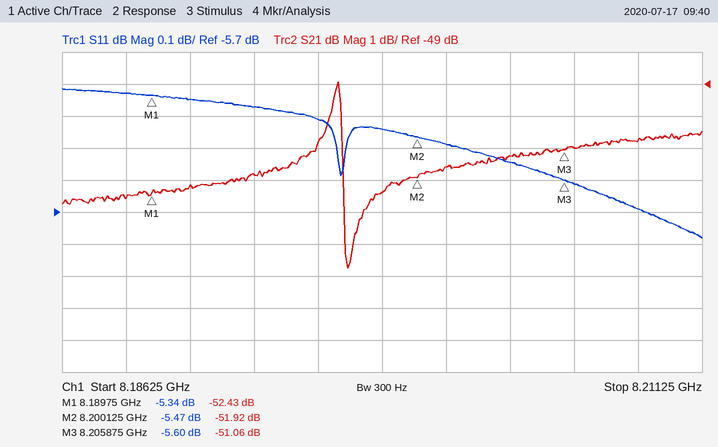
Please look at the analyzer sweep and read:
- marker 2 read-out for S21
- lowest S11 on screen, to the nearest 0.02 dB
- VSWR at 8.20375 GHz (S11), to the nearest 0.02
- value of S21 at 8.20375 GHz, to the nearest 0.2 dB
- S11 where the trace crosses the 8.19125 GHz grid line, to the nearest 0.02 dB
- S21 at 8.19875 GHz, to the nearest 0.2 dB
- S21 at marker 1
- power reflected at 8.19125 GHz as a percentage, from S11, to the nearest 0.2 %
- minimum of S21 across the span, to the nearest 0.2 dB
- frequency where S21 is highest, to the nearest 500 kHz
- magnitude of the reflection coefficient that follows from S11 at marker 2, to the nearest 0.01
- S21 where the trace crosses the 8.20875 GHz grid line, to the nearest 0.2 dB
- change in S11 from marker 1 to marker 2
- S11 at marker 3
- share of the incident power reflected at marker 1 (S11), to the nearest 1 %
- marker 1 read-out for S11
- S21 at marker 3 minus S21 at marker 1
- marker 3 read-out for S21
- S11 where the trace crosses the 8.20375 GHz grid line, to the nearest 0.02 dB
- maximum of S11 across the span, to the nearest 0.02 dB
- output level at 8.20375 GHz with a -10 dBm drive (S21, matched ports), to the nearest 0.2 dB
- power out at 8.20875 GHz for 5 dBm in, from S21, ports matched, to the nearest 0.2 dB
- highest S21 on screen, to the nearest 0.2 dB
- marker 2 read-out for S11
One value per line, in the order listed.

-51.92 dB
-5.78 dB
3.24
-51.2 dB
-5.34 dB
-52.4 dB
-52.43 dB
29.2 %
-54.8 dB
8.1970 GHz
0.53
-50.8 dB
-0.13 dB
-5.60 dB
29 %
-5.34 dB
1.37 dB
-51.06 dB
-5.54 dB
-5.32 dB
-61.2 dBm
-45.8 dBm
-49.0 dB
-5.47 dB
